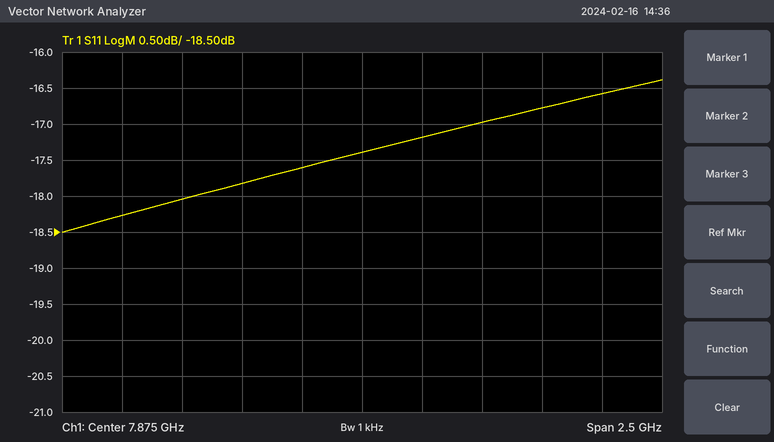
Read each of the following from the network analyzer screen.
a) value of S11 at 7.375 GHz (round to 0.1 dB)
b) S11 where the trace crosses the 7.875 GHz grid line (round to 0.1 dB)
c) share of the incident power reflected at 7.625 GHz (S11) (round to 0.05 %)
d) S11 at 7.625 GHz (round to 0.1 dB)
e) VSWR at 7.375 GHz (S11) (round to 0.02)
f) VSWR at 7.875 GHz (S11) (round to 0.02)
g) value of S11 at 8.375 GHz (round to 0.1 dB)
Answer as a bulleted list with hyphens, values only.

- -17.8 dB
- -17.4 dB
- 1.75 %
- -17.6 dB
- 1.30
- 1.32
- -17.0 dB
